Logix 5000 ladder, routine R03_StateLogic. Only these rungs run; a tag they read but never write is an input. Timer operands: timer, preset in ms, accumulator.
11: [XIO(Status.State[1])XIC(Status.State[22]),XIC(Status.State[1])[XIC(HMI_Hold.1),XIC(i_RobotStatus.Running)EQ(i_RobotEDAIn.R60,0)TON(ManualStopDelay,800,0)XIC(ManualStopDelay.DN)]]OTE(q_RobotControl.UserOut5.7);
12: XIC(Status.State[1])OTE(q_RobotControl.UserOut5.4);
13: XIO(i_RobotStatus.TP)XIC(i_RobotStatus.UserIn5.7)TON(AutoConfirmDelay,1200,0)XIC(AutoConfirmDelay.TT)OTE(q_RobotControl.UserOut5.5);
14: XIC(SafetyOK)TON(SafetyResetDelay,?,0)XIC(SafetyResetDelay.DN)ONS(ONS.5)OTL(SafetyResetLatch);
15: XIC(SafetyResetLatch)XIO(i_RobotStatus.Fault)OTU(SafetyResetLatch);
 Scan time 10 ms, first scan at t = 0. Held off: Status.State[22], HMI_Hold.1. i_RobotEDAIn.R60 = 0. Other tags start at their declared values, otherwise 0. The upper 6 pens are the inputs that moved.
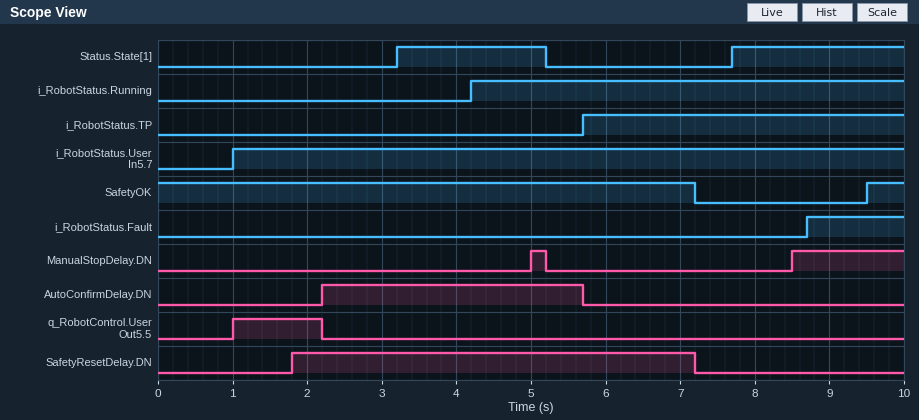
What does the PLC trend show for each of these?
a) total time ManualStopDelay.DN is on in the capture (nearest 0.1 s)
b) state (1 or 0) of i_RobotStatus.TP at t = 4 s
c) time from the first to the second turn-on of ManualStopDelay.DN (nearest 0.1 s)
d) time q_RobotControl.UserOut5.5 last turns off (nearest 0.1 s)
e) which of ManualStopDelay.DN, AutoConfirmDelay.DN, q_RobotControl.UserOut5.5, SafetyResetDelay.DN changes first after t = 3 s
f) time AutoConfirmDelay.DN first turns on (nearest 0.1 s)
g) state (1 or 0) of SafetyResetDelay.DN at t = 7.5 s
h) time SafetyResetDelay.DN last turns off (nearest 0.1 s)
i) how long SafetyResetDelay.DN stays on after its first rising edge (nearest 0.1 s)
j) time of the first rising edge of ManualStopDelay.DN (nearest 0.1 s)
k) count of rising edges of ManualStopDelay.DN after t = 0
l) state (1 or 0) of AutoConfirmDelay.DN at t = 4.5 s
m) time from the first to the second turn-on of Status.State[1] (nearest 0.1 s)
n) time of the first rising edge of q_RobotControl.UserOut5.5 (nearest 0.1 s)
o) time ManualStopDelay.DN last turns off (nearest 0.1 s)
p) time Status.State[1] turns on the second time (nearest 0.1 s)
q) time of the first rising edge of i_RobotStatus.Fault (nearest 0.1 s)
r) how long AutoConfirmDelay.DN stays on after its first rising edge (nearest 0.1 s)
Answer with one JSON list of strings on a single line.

["1.7 s", "0", "3.5 s", "2.2 s", "ManualStopDelay.DN", "2.2 s", "0", "7.2 s", "5.4 s", "5.0 s", "2", "1", "4.5 s", "1.0 s", "5.2 s", "7.7 s", "8.7 s", "3.5 s"]
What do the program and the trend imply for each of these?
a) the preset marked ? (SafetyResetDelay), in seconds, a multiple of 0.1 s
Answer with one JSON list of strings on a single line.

["1.8 s"]
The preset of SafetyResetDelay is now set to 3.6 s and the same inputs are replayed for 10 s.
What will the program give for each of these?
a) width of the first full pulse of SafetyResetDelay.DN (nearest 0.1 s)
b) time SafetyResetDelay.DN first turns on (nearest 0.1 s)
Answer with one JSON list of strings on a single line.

["3.6 s", "3.6 s"]
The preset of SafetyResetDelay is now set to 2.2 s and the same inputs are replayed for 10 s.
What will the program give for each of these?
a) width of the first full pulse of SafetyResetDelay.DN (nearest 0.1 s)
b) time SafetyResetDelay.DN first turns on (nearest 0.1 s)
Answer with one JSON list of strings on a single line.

["5.0 s", "2.2 s"]
